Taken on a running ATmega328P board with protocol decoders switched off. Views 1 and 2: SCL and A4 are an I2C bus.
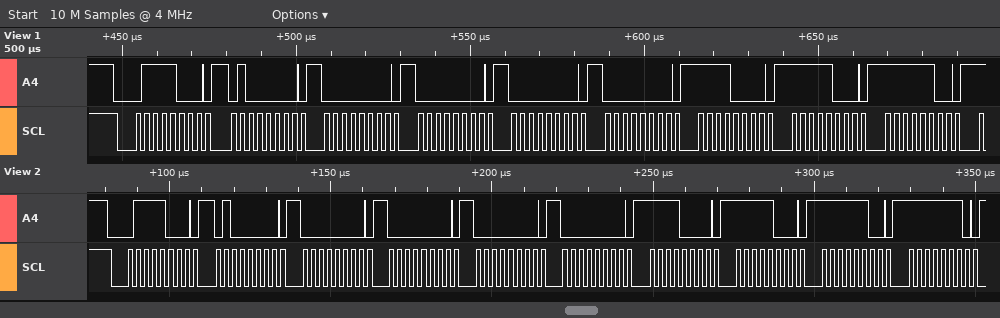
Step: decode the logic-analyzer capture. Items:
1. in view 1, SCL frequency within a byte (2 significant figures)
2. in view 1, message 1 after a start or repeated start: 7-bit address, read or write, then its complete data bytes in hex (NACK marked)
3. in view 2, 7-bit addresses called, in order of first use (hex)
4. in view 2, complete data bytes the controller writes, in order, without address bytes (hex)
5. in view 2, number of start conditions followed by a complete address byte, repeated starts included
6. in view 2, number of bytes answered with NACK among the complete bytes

400 kHz
0x3C write: 40 00 00 00 00 F0 F8 FC
0x3C
40 00 00 00 00 F0 F8 FC FE
1
0
